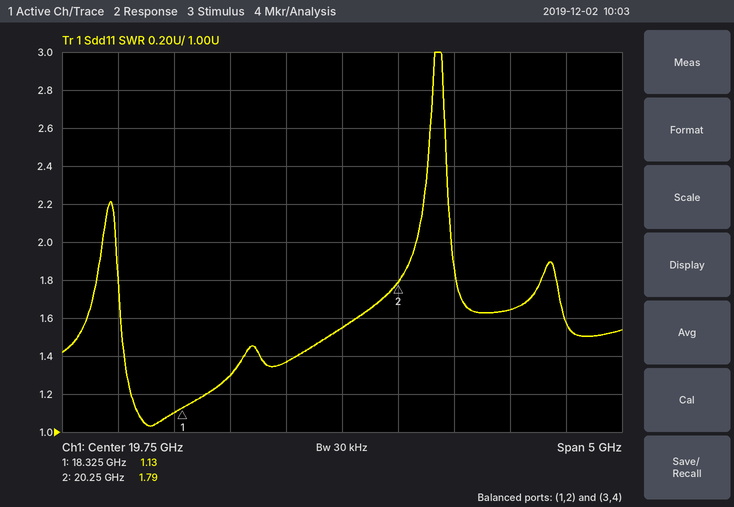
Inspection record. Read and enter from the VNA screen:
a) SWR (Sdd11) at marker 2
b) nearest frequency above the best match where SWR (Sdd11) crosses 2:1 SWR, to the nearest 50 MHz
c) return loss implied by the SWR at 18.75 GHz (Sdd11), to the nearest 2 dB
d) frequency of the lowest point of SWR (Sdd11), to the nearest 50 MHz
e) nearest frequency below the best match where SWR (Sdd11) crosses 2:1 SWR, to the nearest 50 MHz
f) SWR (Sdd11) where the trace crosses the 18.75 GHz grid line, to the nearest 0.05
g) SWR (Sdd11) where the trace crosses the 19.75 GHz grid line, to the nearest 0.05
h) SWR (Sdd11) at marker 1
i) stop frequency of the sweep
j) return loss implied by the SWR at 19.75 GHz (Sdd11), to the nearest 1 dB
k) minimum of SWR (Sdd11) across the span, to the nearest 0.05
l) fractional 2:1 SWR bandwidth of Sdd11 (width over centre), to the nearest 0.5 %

1.79
20.40 GHz
18 dB
18.05 GHz
17.75 GHz
1.30
1.55
1.13
22.25 GHz
13 dB
1.05
14.0 %
